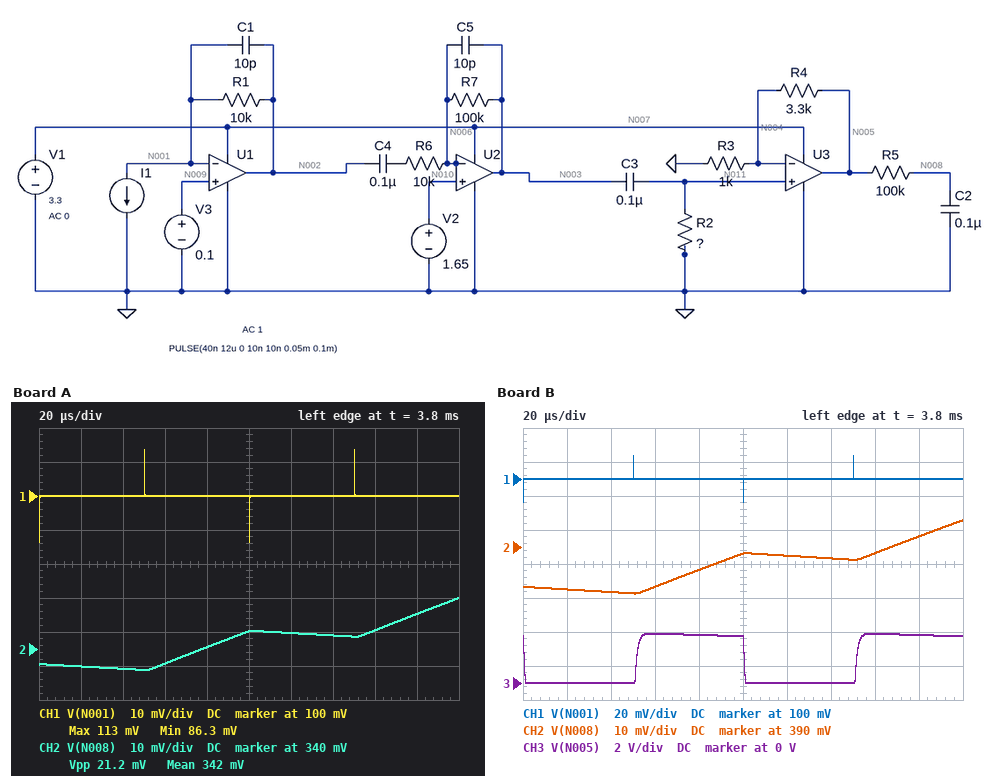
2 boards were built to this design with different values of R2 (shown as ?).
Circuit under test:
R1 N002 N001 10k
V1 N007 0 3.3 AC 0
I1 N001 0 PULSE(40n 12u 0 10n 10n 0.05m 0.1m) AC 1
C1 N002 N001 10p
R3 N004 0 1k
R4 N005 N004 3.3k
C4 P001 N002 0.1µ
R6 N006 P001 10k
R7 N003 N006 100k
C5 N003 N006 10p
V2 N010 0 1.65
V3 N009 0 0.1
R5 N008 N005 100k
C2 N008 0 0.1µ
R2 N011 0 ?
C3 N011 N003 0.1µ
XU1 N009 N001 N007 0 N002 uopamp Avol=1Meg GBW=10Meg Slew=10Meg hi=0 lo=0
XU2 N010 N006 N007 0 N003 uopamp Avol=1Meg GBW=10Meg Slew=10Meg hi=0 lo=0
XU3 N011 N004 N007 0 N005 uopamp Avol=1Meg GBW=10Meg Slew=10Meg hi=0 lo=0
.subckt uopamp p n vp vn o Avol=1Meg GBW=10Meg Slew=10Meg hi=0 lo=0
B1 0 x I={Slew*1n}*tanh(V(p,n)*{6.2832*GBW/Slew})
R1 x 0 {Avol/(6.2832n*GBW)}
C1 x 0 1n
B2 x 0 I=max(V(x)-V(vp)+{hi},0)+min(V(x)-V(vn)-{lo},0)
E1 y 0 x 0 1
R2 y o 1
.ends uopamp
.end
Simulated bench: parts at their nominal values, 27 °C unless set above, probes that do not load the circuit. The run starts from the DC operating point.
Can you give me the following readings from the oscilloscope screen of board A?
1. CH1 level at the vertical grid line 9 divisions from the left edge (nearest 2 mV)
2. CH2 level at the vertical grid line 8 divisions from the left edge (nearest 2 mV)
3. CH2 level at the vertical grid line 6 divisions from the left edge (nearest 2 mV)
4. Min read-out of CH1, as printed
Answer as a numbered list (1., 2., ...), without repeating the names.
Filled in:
1. 100 mV
2. 346 mV
3. 344 mV
4. 86.3 mV
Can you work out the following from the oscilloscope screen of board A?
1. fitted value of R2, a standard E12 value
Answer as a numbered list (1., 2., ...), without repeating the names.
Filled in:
1. 82 kΩ
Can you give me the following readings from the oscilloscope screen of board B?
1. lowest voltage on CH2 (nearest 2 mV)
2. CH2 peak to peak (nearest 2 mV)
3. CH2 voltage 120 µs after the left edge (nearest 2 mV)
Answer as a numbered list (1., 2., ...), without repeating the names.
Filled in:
1. 376 mV
2. 22 mV
3. 388 mV
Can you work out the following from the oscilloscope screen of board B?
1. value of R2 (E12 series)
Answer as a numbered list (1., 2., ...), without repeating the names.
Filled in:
1. 22 kΩ
